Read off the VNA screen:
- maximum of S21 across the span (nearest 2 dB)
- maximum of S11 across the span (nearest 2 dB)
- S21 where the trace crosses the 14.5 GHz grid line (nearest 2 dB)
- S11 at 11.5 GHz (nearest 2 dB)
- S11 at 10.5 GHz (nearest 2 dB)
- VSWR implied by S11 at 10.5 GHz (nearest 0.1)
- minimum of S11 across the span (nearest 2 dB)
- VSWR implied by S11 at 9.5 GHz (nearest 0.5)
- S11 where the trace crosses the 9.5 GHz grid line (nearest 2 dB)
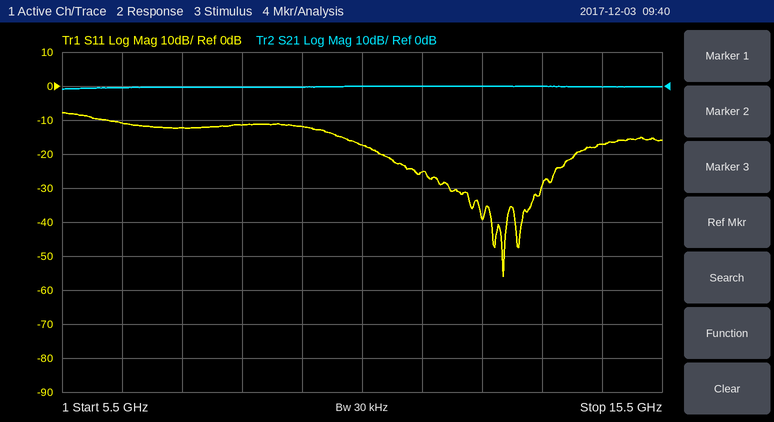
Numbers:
0 dB
-8 dB
0 dB
-26 dB
-18 dB
1.3
-56 dB
1.5
-12 dB
